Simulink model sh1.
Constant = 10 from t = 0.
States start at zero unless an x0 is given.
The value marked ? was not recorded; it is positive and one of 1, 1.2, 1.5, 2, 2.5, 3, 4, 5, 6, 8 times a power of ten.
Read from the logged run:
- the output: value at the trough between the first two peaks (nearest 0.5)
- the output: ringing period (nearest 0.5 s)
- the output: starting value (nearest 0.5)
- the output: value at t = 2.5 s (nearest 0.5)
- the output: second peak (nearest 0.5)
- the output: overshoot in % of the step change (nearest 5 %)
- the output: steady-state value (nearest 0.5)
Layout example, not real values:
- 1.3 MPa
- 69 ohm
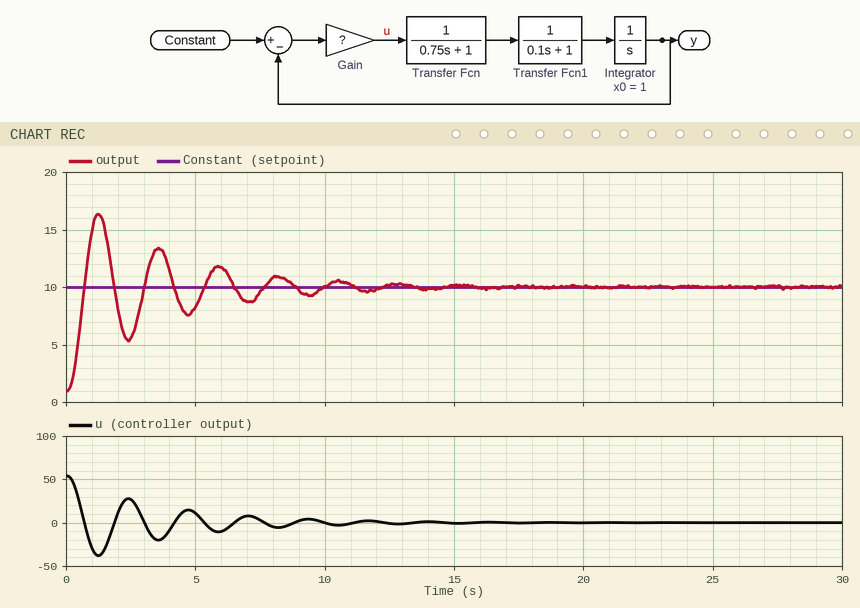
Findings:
- 5.5
- 2.5 s
- 1.0
- 5.5
- 13.5
- 70 %
- 10.0
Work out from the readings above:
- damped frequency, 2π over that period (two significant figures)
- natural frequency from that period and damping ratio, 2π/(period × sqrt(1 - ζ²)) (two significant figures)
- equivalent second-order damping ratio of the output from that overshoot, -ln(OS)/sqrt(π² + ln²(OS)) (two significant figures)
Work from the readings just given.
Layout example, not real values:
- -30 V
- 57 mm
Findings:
- 2.5 rad/s
- 2.5 rad/s
- 0.11
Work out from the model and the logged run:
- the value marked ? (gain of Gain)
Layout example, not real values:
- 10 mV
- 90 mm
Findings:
- 6
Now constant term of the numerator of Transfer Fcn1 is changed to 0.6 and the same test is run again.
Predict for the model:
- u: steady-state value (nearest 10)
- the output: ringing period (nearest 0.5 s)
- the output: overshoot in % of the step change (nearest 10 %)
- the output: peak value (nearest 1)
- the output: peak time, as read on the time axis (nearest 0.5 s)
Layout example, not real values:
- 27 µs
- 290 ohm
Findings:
- 0
- 3.0 s
- 50 %
- 15
- 1.5 s
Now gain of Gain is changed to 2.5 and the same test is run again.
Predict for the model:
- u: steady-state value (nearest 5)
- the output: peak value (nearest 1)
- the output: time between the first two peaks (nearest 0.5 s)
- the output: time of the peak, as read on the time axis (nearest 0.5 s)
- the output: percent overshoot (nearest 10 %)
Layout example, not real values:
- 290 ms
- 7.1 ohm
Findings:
- 0
- 14
- 3.5 s
- 2.0 s
- 40 %
